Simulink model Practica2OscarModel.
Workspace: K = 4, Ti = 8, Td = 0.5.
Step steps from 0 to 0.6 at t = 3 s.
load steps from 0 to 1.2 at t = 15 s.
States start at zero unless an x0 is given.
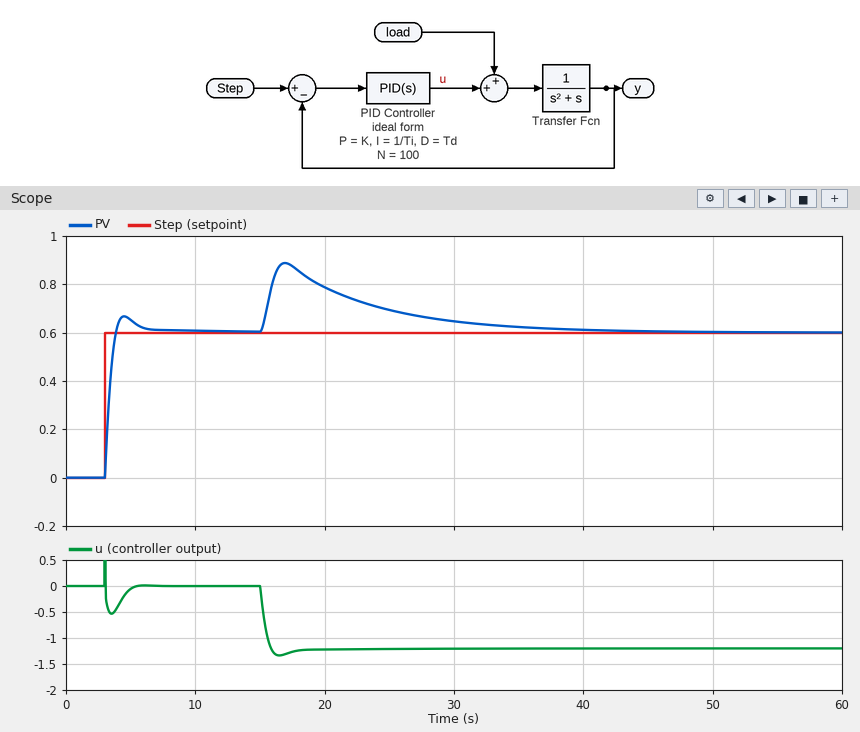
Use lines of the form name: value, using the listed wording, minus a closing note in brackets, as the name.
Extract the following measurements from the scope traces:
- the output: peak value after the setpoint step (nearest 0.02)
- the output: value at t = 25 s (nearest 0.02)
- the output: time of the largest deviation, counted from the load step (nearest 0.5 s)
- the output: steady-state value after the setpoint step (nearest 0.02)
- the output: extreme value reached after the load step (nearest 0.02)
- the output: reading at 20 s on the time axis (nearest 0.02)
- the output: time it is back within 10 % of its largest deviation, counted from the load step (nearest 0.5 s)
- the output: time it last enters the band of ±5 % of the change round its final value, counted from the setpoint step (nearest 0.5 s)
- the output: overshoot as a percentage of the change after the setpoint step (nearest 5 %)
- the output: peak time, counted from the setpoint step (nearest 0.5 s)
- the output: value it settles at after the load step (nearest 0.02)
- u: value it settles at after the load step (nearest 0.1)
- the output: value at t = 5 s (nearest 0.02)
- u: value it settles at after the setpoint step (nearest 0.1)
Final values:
the output: peak value after the setpoint step: 0.66
the output: value at t = 25 s: 0.70
the output: time of the largest deviation, counted from the load step: 2.0 s
the output: steady-state value after the setpoint step: 0.60
the output: extreme value reached after the load step: 0.88
the output: reading at 20 s on the time axis: 0.78
the output: time it is back within 10 % of its largest deviation, counted from the load step: 18.5 s
the output: time it last enters the band of ±5 % of the change round its final value, counted from the setpoint step: 2.5 s
the output: overshoot as a percentage of the change after the setpoint step: 10 %
the output: peak time, counted from the setpoint step: 1.5 s
the output: value it settles at after the load step: 0.60
u: value it settles at after the load step: -1.2
the output: value at t = 5 s: 0.66
u: value it settles at after the setpoint step: 0.0
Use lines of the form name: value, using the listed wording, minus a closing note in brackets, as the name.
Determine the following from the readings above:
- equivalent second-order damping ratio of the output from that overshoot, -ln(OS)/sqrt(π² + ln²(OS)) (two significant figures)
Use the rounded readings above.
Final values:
equivalent second-order damping ratio of the output from that overshoot, -ln(OS)/sqrt(π² + ln²(OS)): 0.59
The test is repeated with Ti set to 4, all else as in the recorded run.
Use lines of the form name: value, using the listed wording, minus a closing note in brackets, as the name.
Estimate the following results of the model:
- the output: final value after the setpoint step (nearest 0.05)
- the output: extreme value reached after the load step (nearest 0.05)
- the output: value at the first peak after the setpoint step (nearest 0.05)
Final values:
the output: final value after the setpoint step: 0.60
the output: extreme value reached after the load step: 0.85
the output: value at the first peak after the setpoint step: 0.70
